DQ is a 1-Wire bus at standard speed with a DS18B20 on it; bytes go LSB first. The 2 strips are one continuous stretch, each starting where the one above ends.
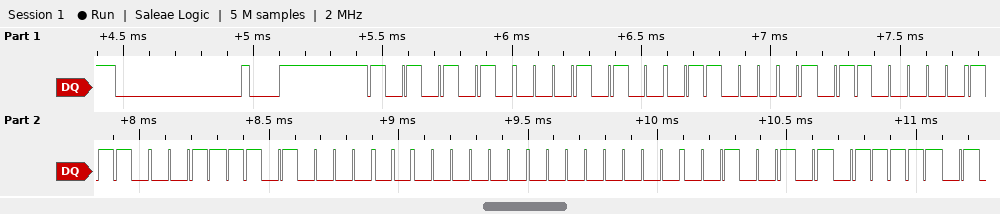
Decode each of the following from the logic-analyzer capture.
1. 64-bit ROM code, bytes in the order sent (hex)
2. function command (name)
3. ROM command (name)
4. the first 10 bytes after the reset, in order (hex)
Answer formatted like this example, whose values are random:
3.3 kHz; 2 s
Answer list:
28 86 06 C7 0B 00 00 A4; Read Scratchpad; Match ROM; 55 28 86 06 C7 0B 00 00 A4 BE
